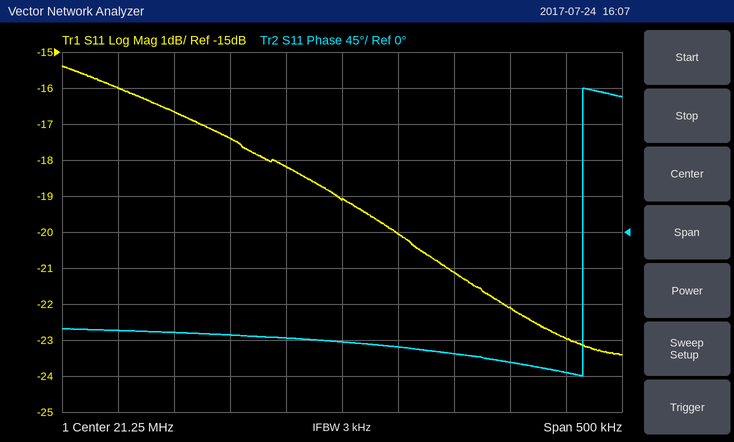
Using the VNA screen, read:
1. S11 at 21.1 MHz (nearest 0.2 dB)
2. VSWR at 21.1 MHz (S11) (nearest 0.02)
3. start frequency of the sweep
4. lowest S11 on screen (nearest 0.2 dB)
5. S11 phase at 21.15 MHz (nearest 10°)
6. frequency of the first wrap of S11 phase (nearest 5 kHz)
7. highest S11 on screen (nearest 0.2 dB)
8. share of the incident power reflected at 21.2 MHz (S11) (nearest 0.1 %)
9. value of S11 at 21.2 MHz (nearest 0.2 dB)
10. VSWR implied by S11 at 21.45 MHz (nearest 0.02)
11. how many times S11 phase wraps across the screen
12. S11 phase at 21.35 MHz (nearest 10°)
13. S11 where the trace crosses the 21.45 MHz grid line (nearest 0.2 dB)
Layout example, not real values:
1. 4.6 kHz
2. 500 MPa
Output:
1. -16.6 dB
2. 1.34
3. 21 MHz
4. -23.4 dB
5. -130°
6. 21.465 MHz
7. -15.4 dB
8. 1.5 %
9. -18.2 dB
10. 1.16
11. 1
12. -150°
13. -23.0 dB
